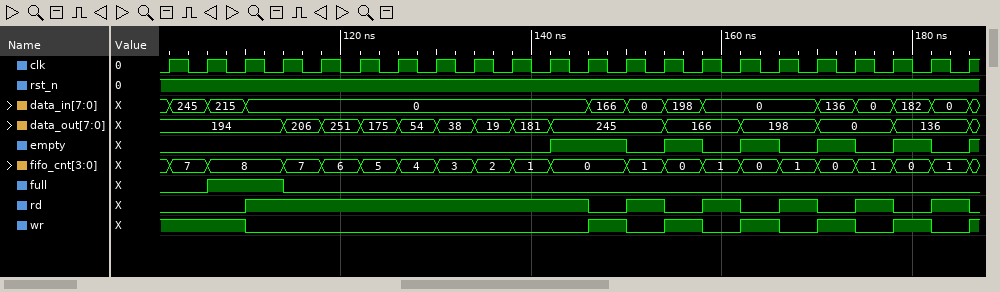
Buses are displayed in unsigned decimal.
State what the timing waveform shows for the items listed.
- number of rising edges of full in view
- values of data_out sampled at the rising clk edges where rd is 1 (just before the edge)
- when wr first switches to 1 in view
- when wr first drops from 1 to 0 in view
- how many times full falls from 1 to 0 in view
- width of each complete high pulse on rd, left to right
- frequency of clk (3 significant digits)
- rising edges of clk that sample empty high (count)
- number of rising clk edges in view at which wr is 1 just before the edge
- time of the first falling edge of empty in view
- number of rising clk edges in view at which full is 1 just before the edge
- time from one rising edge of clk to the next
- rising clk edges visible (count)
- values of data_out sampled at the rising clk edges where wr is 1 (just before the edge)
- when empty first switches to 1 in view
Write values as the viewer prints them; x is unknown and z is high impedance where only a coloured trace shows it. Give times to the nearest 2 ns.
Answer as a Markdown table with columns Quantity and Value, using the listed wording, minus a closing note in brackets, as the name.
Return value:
| Quantity | Value |
|---|---|
| number of rising edges of full in view | 1 |
| values of data_out sampled at the rising clk edges where rd is 1 | 194, 206, 251, 175, 54, 38, 19, 181, 245, 245, 166, 198, 0, 136 |
| when wr first switches to 1 in view | 146 ns |
| when wr first drops from 1 to 0 in view | 110 ns |
| how many times full falls from 1 to 0 in view | 1 |
| width of each complete high pulse on rd, left to right | 36 ns, 4 ns, 4 ns, 4 ns, 4 ns, 4 ns |
| frequency of clk | 250 MHz |
| rising edges of clk that sample empty high | 6 |
| number of rising clk edges in view at which wr is 1 just before the edge | 8 |
| time of the first falling edge of empty in view | 150 ns |
| number of rising clk edges in view at which full is 1 just before the edge | 2 |
| time from one rising edge of clk to the next | 4 ns |
| rising clk edges visible | 22 |
| values of data_out sampled at the rising clk edges where wr is 1 | 194, 194, 194, 245, 166, 198, 0, 136 |
| when empty first switches to 1 in view | 142 ns |
